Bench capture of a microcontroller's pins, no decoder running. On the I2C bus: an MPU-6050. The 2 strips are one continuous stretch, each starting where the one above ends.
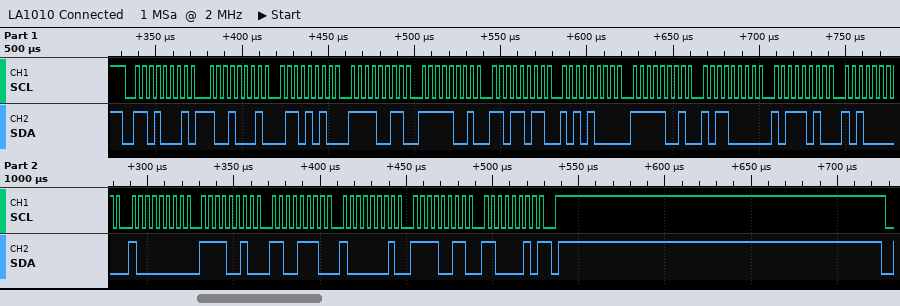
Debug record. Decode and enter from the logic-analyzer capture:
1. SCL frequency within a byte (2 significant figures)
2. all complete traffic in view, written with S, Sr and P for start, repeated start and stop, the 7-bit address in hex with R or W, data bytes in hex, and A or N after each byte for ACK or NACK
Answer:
250 kHz
S 68R A 91 A 6A A F3 A F9 A DB A A8 A F9 A B0 A BA A A0 A 80 A F2 A CE A 81 A F3 A C2 N P
